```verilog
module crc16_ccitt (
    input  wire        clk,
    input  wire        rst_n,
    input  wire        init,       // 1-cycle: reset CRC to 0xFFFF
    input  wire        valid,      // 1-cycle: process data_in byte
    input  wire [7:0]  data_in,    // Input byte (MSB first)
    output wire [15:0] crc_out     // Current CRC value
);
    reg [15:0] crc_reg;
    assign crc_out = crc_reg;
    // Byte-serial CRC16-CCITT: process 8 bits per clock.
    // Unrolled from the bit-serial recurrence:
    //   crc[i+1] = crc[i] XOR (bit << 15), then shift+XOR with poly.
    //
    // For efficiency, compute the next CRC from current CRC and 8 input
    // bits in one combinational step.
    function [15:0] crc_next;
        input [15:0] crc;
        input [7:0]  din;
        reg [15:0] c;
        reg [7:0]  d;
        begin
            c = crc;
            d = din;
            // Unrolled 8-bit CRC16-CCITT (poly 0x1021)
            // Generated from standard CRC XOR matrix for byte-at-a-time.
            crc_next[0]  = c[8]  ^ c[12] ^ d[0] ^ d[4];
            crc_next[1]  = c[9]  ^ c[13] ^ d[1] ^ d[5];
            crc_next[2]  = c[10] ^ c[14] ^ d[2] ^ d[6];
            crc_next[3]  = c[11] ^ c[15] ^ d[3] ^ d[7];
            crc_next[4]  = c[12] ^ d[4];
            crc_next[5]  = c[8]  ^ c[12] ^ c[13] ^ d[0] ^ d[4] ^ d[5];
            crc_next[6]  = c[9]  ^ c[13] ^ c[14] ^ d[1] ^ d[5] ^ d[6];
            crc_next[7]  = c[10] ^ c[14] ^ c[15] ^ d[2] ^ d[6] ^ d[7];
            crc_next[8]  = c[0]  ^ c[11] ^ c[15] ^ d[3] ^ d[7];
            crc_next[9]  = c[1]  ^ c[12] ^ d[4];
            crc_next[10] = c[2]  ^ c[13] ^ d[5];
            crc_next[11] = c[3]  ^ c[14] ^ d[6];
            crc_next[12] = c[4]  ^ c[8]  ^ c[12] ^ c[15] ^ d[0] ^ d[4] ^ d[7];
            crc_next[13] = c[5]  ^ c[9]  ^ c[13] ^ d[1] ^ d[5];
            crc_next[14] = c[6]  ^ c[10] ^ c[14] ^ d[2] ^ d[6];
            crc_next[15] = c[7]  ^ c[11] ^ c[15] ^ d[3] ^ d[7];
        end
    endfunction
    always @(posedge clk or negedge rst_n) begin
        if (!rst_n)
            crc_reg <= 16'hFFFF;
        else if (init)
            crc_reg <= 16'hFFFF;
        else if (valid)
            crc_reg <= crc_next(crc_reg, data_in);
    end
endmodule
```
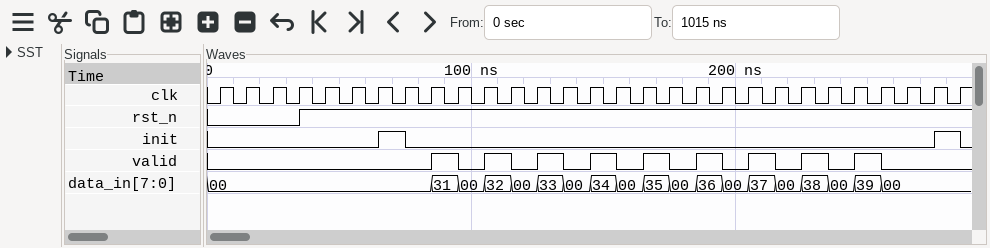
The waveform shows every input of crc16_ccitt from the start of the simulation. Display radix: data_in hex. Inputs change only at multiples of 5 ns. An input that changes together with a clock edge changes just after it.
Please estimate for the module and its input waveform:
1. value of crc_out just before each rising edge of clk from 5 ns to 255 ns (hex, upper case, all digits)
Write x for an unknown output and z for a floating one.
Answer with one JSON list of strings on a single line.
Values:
["FFFF, FFFF, FFFF, FFFF, FFFF, FFFF, FFFF, FFFF, FFFF, FFFF, C782, C782, 3DBA, 3DBA, 5BCE, 5BCE, 5349, 5349, 4560, 4560, 2EF4, 2EF4, 7718, 7718, A12B, A12B"]
